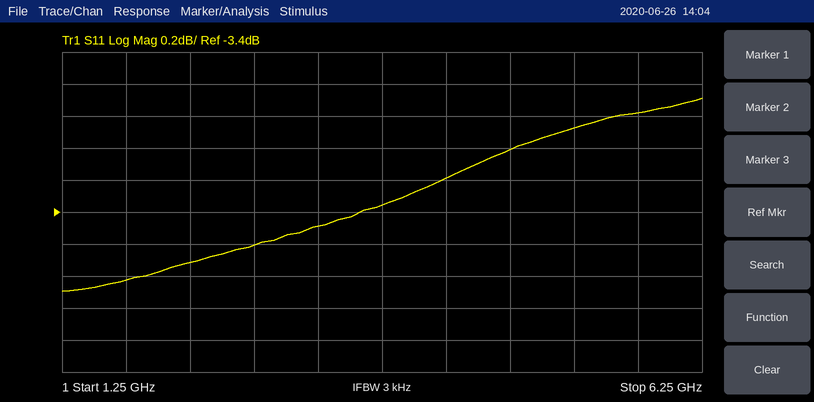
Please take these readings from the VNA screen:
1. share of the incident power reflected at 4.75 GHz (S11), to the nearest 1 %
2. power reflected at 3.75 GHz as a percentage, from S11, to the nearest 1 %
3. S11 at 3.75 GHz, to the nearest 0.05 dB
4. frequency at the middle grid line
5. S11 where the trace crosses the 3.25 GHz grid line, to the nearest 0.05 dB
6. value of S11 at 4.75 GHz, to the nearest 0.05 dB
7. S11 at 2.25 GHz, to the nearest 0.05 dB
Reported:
50 %
46 %
-3.35 dB
3.75 GHz
-3.50 dB
-3.00 dB
-3.70 dB
